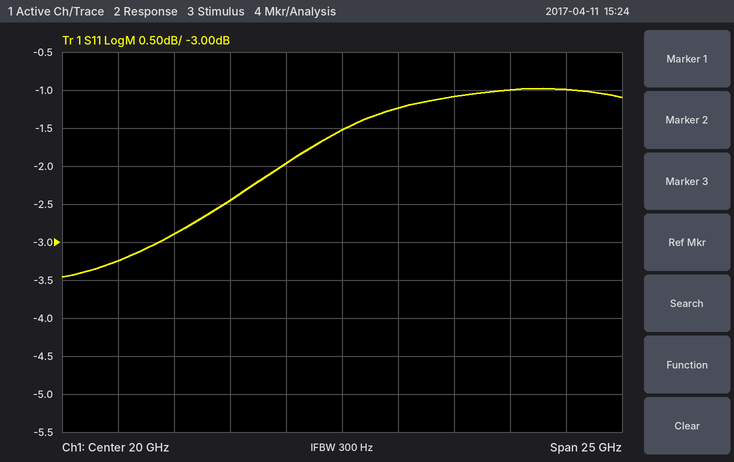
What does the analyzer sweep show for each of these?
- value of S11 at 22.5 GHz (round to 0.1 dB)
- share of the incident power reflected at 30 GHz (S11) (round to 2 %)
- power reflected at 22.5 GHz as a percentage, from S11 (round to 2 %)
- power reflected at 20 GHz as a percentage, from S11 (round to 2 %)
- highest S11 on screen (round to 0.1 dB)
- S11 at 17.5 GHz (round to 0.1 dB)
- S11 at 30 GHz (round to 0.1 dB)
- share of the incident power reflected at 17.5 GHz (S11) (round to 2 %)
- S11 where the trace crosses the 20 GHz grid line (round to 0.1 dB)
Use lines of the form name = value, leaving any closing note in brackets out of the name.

value of S11 at 22.5 GHz = -1.2 dB
share of the incident power reflected at 30 GHz (S11) = 80 %
power reflected at 22.5 GHz as a percentage, from S11 = 76 %
power reflected at 20 GHz as a percentage, from S11 = 70 %
highest S11 on screen = -1.0 dB
S11 at 17.5 GHz = -2.0 dB
S11 at 30 GHz = -1.0 dB
share of the incident power reflected at 17.5 GHz (S11) = 64 %
S11 where the trace crosses the 20 GHz grid line = -1.5 dB
